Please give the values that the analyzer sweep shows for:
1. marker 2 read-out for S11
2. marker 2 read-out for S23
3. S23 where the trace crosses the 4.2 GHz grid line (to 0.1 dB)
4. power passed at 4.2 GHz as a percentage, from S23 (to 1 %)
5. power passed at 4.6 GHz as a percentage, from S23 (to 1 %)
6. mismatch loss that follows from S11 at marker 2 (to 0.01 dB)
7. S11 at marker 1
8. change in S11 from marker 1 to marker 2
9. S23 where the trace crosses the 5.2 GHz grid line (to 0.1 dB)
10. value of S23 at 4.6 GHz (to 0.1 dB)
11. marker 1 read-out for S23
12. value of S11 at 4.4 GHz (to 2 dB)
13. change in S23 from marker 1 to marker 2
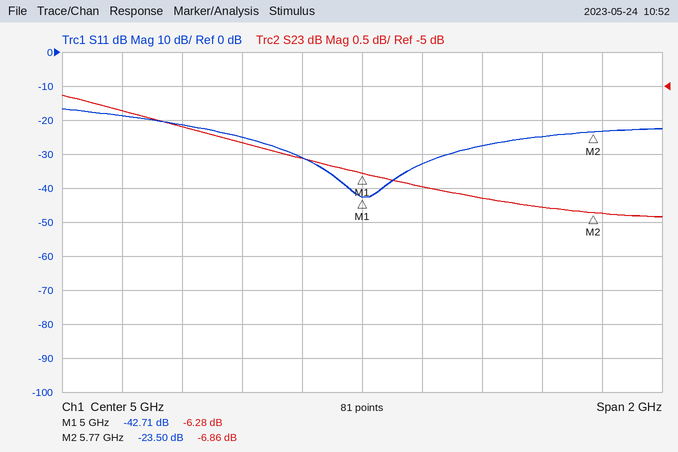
-23.50 dB
-6.86 dB
-5.4 dB
29 %
26 %
0.02 dB
-42.71 dB
19.21 dB
-6.5 dB
-5.8 dB
-6.28 dB
-22 dB
-0.58 dB
